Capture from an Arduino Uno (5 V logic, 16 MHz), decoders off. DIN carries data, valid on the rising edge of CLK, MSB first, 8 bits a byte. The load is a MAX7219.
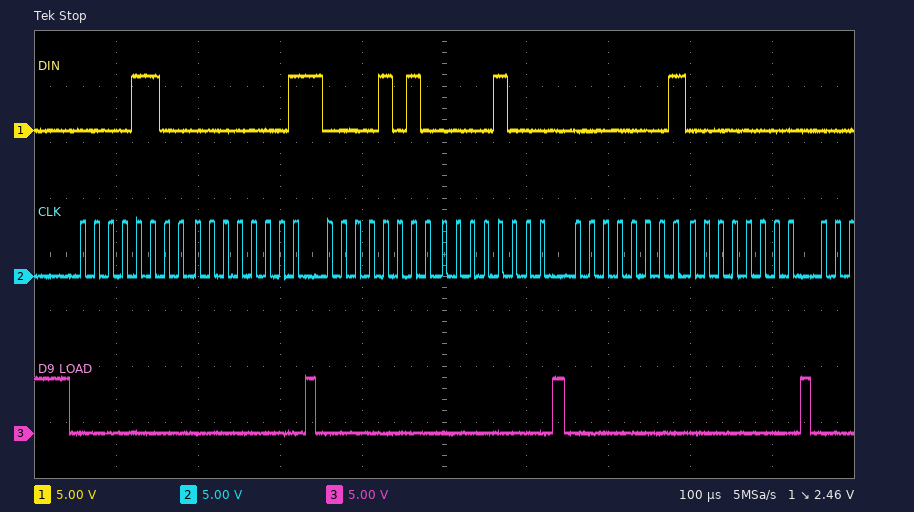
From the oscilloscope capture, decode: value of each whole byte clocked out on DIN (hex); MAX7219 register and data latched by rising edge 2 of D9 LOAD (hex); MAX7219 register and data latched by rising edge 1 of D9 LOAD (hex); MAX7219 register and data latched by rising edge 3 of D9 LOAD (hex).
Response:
0C 01 0A 08 01 00
register 0xA, data 0x08
register 0xC, data 0x01
register 0x1, data 0x00
